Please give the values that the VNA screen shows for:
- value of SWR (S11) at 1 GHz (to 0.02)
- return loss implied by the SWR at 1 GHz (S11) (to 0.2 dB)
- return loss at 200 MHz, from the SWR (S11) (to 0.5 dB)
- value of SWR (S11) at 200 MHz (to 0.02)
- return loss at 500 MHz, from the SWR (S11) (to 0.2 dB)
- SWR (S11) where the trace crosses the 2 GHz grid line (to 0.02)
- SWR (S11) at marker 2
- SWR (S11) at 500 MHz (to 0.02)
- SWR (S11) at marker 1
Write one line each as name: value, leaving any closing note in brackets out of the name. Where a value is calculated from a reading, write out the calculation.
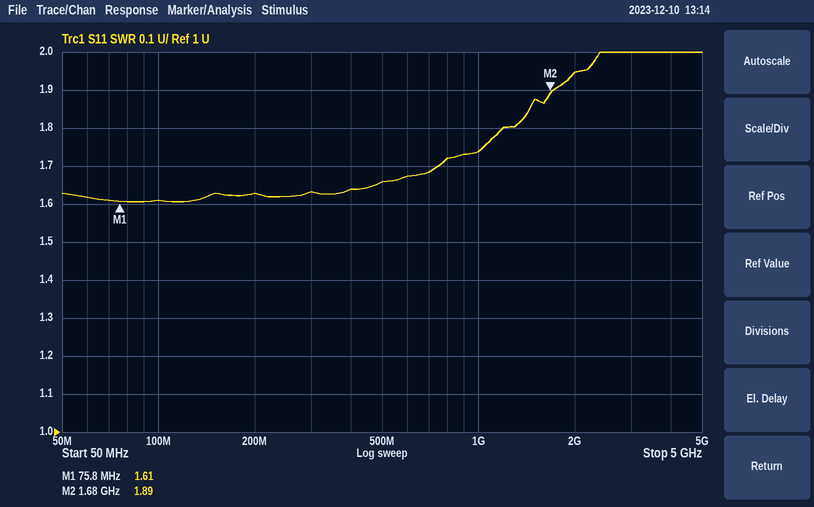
value of SWR (S11) at 1 GHz: 1.74
return loss implied by the SWR at 1 GHz (S11): −20 log10((1.74 − 1)/(1.74 + 1)) ≈ 11.4 dB
return loss at 200 MHz, from the SWR (S11): −20 log10((1.62 − 1)/(1.62 + 1)) ≈ 12.5 dB
value of SWR (S11) at 200 MHz: 1.62
return loss at 500 MHz, from the SWR (S11): −20 log10((1.66 − 1)/(1.66 + 1)) ≈ 12.1 dB, so 12.2 dB to the nearest 0.2 dB
SWR (S11) where the trace crosses the 2 GHz grid line: 1.94
SWR (S11) at marker 2: 1.89
SWR (S11) at 500 MHz: 1.66
SWR (S11) at marker 1: 1.61
